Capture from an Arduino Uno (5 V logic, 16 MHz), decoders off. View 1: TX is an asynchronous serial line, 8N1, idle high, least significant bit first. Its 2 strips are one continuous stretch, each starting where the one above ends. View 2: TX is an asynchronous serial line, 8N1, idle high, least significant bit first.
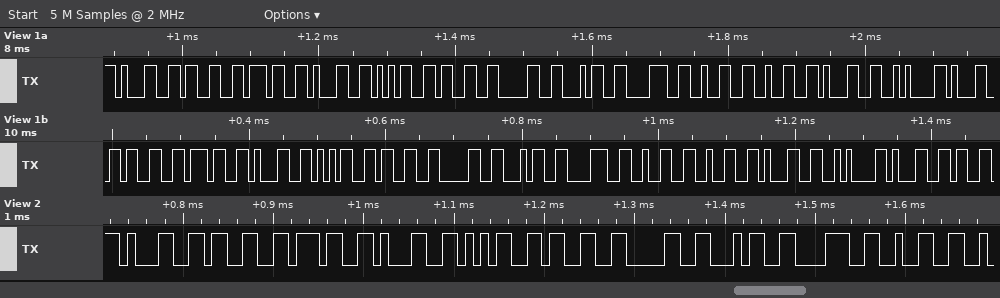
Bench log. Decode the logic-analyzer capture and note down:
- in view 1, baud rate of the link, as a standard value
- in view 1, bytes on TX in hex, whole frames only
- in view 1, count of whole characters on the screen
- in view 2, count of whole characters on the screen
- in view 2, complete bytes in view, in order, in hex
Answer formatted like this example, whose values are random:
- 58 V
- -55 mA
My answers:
- 115200 baud
- 31 33 37 31 35 33 30 34 38 32 32 31 0A 31 33 37 31 35 33 30 34 38 32 32 31 0A 31
- 27
- 10
- 0x31 0x33 0x37 0x31 0x35 0x33 0x30 0x34 0x38 0x32
